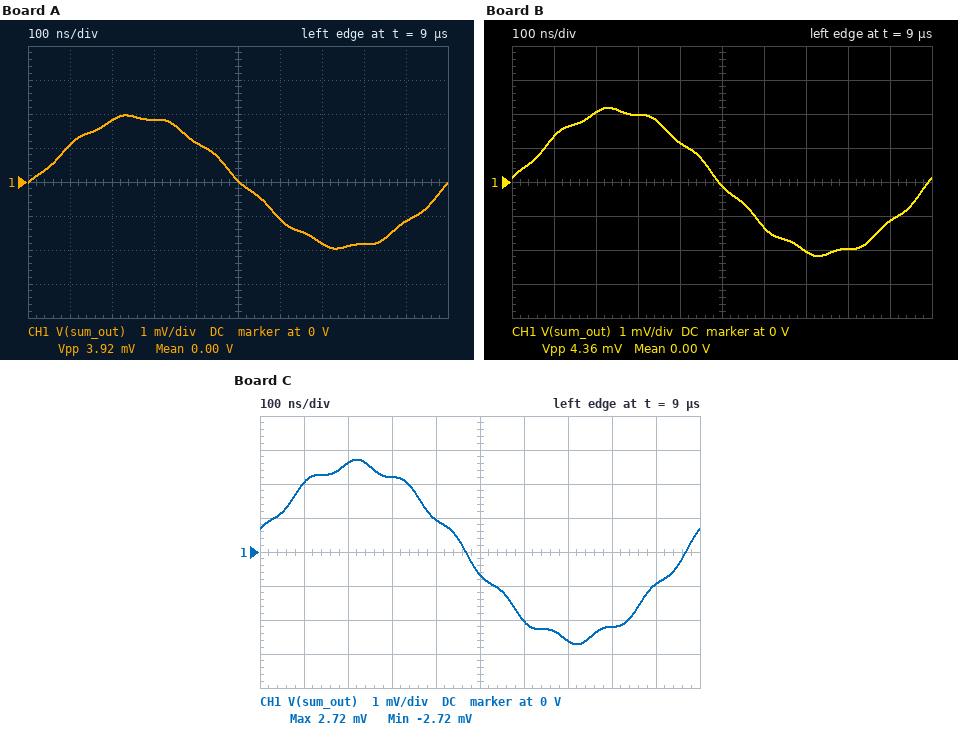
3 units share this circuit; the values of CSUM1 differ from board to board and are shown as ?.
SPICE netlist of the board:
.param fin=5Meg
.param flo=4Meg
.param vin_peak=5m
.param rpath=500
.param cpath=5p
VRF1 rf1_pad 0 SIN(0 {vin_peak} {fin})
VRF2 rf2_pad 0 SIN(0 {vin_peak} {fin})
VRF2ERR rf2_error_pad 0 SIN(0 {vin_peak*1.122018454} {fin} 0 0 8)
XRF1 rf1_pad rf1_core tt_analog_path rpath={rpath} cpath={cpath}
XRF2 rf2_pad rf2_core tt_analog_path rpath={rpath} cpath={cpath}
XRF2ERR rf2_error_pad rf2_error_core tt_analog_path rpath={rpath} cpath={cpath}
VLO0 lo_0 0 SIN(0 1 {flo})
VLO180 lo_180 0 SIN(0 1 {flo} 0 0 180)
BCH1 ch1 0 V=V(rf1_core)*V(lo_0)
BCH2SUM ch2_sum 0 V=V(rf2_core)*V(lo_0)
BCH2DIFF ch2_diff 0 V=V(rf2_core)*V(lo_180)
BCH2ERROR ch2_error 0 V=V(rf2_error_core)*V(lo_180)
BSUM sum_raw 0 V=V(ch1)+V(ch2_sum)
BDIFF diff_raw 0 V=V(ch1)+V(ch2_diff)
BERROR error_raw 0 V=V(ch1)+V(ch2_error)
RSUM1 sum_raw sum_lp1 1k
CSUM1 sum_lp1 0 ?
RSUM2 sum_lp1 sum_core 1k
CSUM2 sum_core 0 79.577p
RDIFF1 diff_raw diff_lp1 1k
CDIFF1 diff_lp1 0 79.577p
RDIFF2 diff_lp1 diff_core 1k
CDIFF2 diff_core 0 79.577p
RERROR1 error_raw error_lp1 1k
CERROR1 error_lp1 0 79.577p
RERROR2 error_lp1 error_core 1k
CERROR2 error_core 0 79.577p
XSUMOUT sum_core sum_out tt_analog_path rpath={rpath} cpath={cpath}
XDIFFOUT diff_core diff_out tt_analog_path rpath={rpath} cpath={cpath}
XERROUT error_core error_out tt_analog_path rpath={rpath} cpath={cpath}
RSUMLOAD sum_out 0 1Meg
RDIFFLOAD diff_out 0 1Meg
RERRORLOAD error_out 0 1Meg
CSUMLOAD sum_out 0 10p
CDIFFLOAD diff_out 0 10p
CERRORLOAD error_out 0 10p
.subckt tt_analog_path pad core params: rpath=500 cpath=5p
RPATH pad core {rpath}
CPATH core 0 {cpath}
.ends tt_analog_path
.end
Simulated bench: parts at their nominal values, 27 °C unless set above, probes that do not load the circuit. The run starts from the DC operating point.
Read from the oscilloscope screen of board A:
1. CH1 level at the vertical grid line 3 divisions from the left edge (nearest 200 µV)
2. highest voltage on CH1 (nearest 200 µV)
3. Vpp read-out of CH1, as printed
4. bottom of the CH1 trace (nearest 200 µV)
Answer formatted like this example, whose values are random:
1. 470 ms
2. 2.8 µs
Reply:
1. 1.8 mV
2. 2.0 mV
3. 3.92 mV
4. -2.0 mV
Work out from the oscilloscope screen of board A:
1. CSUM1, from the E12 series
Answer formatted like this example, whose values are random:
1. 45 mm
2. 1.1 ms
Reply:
1. 220 pF
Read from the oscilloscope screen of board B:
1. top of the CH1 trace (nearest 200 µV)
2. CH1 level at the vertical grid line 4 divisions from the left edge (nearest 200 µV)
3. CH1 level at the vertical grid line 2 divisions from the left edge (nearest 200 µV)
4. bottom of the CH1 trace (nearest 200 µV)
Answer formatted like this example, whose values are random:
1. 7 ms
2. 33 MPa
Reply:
1. 2.2 mV
2. 1.2 mV
3. 2.0 mV
4. -2.2 mV
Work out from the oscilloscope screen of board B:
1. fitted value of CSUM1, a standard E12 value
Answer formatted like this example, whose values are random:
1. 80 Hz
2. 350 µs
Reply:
1. 180 pF
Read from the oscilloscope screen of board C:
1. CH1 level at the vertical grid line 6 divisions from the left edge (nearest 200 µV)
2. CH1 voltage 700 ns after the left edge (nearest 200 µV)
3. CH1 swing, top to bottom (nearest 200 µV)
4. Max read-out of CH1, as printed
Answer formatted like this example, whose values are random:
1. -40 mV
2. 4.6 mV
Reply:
1. -2.0 mV
2. -2.6 mV
3. 5.4 mV
4. 2.72 mV
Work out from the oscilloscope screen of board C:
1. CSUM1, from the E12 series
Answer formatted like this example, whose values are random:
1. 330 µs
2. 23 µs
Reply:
1. 100 pF
